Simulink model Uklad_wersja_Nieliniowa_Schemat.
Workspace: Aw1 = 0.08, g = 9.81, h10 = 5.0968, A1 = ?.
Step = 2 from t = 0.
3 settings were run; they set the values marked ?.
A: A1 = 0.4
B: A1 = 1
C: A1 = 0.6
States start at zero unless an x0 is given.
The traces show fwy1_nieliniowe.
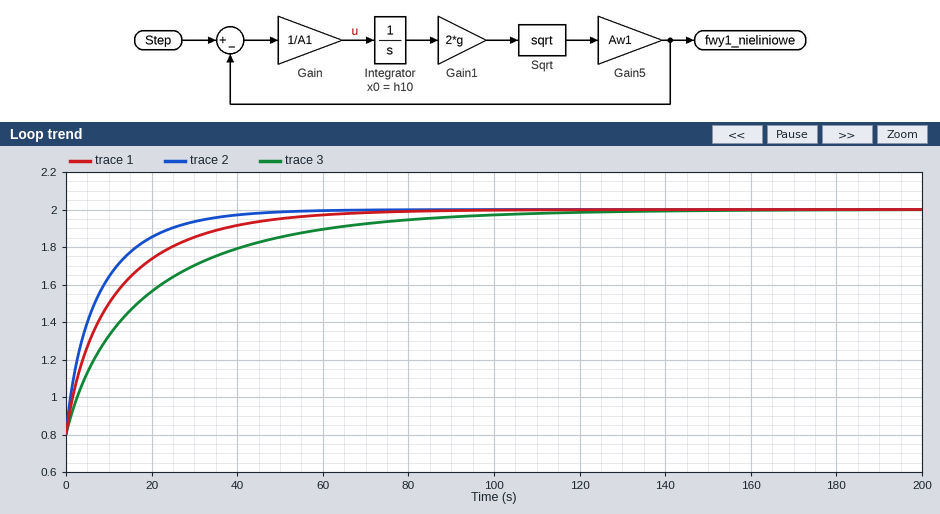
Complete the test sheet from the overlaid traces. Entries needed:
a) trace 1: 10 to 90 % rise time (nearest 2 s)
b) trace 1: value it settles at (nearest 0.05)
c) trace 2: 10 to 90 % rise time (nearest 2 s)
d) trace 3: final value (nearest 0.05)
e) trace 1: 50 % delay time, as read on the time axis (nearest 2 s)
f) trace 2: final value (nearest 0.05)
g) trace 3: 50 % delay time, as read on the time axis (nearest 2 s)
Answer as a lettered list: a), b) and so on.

a) 32 s
b) 2.00
c) 22 s
d) 2.00
e) 8 s
f) 2.00
g) 12 s
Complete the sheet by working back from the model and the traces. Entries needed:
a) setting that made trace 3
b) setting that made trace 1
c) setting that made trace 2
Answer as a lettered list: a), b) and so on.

a) B
b) C
c) A
